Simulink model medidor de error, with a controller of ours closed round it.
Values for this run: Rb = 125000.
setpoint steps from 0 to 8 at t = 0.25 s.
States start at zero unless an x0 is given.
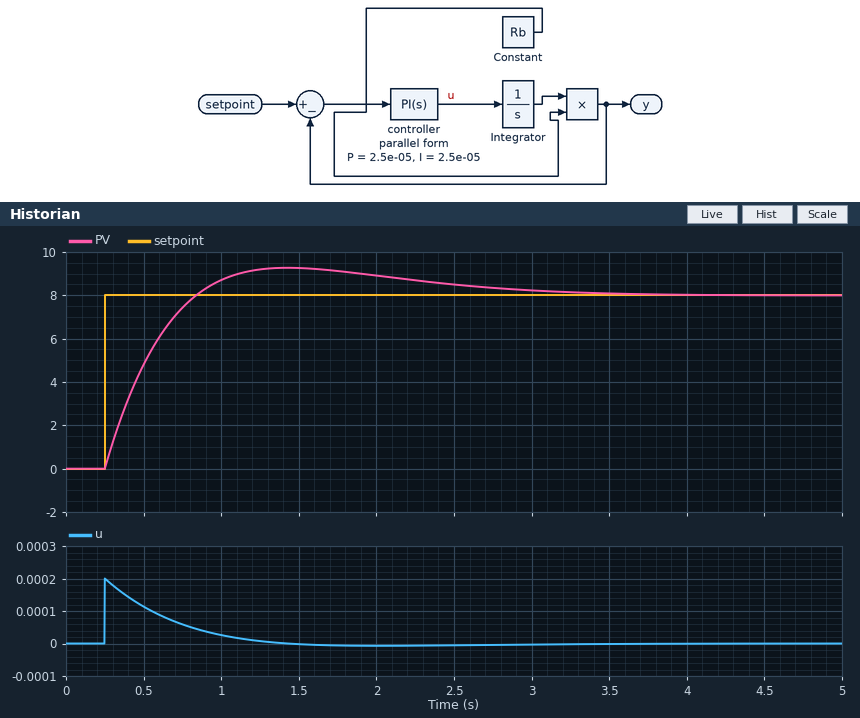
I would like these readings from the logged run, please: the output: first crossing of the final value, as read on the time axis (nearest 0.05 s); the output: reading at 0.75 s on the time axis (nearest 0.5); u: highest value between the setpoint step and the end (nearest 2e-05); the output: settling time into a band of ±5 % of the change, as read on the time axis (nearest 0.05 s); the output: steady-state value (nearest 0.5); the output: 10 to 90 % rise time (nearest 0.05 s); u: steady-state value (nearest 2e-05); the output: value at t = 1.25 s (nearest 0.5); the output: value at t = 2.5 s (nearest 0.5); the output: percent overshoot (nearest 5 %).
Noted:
0.85 s
7.5
0.00020
2.65 s
8.0
0.45 s
0.00000
9.0
8.5
15 %
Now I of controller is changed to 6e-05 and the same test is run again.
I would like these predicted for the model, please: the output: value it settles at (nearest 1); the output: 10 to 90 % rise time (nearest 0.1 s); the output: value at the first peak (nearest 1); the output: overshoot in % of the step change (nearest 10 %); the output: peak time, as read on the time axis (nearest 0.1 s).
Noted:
8
0.3 s
10
30 %
1.1 s
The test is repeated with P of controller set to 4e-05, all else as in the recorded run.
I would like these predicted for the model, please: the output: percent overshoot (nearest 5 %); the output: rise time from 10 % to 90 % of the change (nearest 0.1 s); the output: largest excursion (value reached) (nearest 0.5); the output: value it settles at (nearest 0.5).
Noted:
10 %
0.3 s
8.5
8.0
